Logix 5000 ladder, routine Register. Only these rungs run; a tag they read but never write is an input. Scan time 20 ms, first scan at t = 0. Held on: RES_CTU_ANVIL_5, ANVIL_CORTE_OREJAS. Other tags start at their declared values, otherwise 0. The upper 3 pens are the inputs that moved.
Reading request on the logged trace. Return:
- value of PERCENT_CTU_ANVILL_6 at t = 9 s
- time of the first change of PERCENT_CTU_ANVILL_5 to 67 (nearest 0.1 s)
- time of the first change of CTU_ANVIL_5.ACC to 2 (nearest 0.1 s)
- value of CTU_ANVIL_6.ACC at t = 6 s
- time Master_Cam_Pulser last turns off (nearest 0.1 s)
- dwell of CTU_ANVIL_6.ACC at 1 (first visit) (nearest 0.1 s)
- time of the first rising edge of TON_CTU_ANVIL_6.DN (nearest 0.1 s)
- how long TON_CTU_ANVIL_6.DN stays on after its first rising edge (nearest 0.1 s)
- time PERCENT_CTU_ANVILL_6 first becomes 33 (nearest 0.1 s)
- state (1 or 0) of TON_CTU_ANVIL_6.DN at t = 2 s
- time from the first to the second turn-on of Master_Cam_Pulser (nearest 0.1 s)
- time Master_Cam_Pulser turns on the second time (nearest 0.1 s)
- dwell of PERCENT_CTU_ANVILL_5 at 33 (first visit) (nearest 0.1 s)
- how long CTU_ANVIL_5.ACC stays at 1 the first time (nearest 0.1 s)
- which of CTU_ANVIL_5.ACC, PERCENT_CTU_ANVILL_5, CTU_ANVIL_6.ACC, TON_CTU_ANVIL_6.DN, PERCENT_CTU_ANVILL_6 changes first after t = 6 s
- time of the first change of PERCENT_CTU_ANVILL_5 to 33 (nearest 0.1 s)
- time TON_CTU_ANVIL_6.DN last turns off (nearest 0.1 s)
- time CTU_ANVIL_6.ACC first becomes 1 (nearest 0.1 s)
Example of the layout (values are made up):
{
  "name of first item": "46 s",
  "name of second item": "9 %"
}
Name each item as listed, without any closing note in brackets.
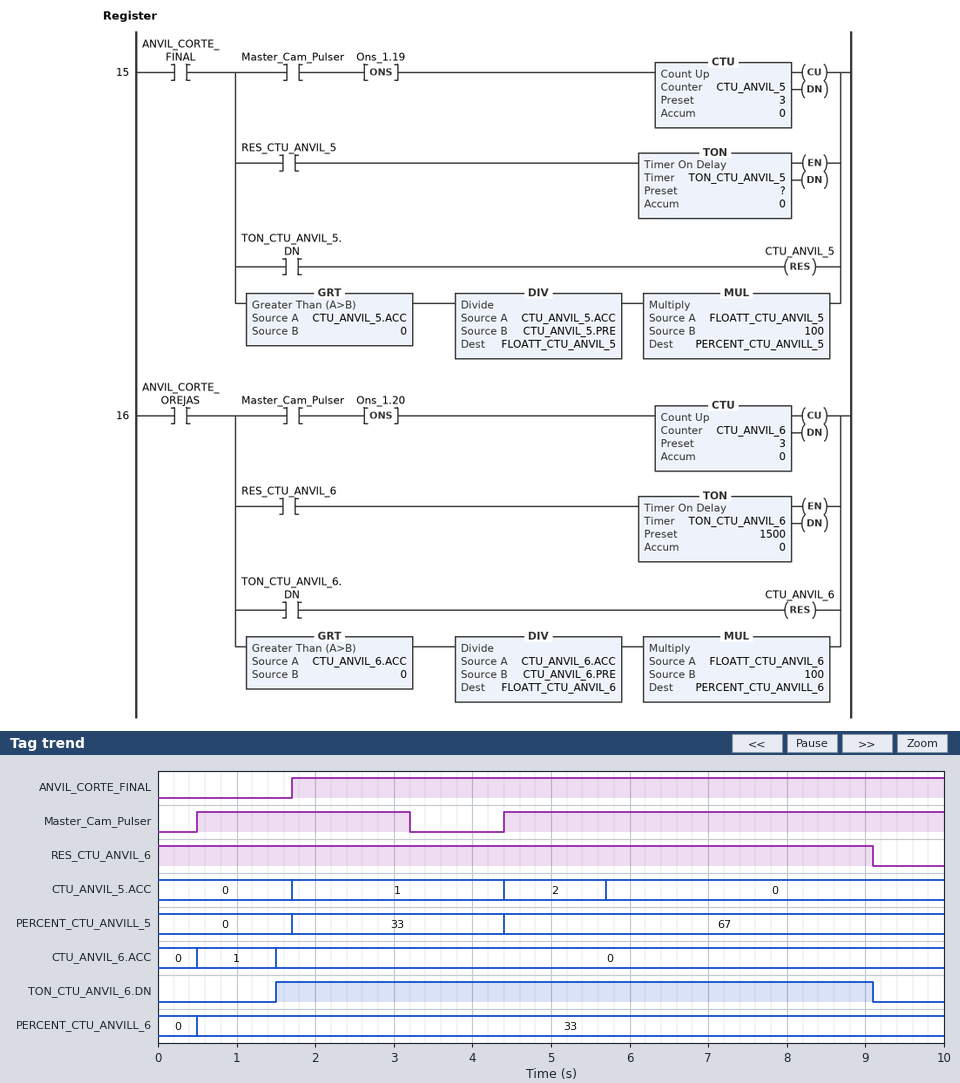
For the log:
{
  "value of PERCENT_CTU_ANVILL_6 at t = 9 s": "33",
  "time of the first change of PERCENT_CTU_ANVILL_5 to 67": "4.4 s",
  "time of the first change of CTU_ANVIL_5.ACC to 2": "4.4 s",
  "value of CTU_ANVIL_6.ACC at t = 6 s": "0",
  "time Master_Cam_Pulser last turns off": "3.2 s",
  "dwell of CTU_ANVIL_6.ACC at 1 (first visit)": "1.0 s",
  "time of the first rising edge of TON_CTU_ANVIL_6.DN": "1.5 s",
  "how long TON_CTU_ANVIL_6.DN stays on after its first rising edge": "7.6 s",
  "time PERCENT_CTU_ANVILL_6 first becomes 33": "0.5 s",
  "state (1 or 0) of TON_CTU_ANVIL_6.DN at t = 2 s": "1",
  "time from the first to the second turn-on of Master_Cam_Pulser": "3.9 s",
  "time Master_Cam_Pulser turns on the second time": "4.4 s",
  "dwell of PERCENT_CTU_ANVILL_5 at 33 (first visit)": "2.7 s",
  "how long CTU_ANVIL_5.ACC stays at 1 the first time": "2.7 s",
  "which of CTU_ANVIL_5.ACC, PERCENT_CTU_ANVILL_5, CTU_ANVIL_6.ACC, TON_CTU_ANVIL_6.DN, PERCENT_CTU_ANVILL_6 changes first after t = 6 s": "TON_CTU_ANVIL_6.DN",
  "time of the first change of PERCENT_CTU_ANVILL_5 to 33": "1.7 s",
  "time TON_CTU_ANVIL_6.DN last turns off": "9.1 s",
  "time CTU_ANVIL_6.ACC first becomes 1": "0.5 s"
}
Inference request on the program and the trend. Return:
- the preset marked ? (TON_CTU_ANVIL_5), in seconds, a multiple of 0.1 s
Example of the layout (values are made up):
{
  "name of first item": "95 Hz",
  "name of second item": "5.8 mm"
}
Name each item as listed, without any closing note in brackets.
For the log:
{
  "the preset marked ? (TON_CTU_ANVIL_5), in seconds, a multiple of 0.1 s": "4.0 s"
}
